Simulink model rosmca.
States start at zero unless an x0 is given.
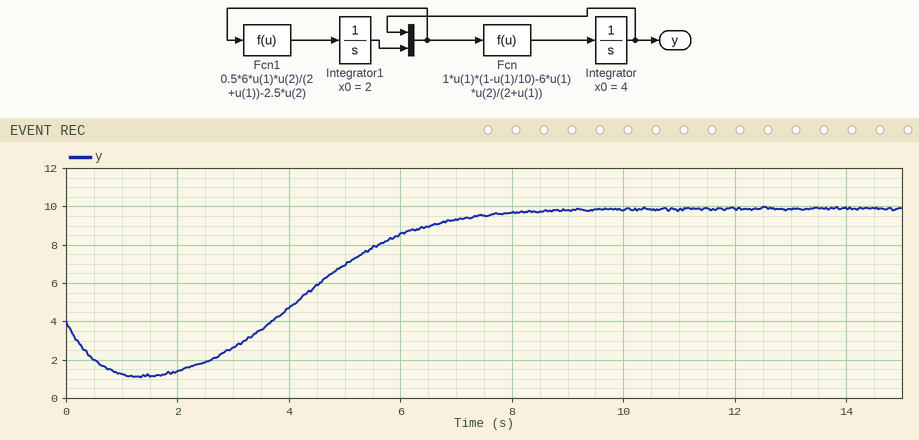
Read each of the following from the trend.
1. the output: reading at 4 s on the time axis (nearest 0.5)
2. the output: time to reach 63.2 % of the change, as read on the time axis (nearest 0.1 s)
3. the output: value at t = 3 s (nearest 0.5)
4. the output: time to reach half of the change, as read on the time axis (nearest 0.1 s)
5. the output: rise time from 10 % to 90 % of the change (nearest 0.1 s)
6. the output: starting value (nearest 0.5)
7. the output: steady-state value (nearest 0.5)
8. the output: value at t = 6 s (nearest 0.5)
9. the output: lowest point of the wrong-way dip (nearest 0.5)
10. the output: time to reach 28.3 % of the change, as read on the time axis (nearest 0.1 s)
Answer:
4.5
5.4 s
2.5
5.0 s
3.1 s
4.0
10.0
8.5
1.0
4.4 s
